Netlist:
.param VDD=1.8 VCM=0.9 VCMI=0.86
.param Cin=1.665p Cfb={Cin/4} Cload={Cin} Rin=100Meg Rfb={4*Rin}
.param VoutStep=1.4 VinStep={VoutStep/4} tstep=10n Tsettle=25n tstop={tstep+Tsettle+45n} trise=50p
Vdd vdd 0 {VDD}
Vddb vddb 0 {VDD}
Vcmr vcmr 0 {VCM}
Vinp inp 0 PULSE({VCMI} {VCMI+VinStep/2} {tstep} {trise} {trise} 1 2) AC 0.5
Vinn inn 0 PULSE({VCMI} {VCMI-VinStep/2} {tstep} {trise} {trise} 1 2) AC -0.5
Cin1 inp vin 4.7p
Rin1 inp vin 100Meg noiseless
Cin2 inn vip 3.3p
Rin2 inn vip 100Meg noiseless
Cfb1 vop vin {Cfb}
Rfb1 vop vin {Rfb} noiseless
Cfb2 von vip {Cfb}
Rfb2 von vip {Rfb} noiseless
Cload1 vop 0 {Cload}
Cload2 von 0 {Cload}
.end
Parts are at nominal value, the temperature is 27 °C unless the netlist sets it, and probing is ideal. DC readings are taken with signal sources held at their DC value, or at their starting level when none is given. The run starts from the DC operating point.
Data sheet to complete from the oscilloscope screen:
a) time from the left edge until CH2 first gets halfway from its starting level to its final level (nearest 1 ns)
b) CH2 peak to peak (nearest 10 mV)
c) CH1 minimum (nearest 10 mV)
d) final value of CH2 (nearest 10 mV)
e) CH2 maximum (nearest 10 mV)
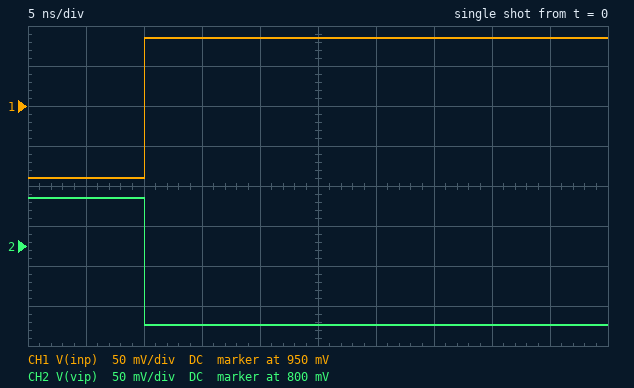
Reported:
10 ns
160 mV
860 mV
700 mV
860 mV
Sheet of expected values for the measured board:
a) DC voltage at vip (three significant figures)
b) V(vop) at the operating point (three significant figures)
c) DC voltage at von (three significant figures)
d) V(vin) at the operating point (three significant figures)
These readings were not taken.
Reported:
860 mV
860 mV
860 mV
860 mV
